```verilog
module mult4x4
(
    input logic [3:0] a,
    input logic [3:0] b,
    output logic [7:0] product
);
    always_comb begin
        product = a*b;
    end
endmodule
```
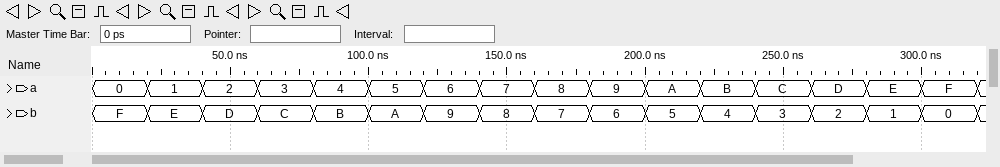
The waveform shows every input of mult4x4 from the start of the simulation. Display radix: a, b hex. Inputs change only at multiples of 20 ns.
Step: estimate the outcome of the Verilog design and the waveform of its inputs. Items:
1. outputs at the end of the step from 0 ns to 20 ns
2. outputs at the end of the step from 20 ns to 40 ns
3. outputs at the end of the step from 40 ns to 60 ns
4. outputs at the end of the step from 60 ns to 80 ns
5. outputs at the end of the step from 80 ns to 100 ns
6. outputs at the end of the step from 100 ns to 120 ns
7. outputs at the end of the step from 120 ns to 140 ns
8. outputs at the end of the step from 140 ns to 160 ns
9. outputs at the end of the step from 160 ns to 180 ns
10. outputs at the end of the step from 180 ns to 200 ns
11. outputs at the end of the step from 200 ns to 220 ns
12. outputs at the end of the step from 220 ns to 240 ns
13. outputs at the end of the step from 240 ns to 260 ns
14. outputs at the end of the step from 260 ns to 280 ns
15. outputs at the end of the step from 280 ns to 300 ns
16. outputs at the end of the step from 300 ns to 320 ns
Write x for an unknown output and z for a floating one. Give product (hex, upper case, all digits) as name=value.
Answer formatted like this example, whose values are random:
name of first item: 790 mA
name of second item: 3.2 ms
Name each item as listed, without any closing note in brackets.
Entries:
outputs at the end of the step from 0 ns to 20 ns: product=00
outputs at the end of the step from 20 ns to 40 ns: product=0E
outputs at the end of the step from 40 ns to 60 ns: product=1A
outputs at the end of the step from 60 ns to 80 ns: product=24
outputs at the end of the step from 80 ns to 100 ns: product=2C
outputs at the end of the step from 100 ns to 120 ns: product=32
outputs at the end of the step from 120 ns to 140 ns: product=36
outputs at the end of the step from 140 ns to 160 ns: product=38
outputs at the end of the step from 160 ns to 180 ns: product=38
outputs at the end of the step from 180 ns to 200 ns: product=36
outputs at the end of the step from 200 ns to 220 ns: product=32
outputs at the end of the step from 220 ns to 240 ns: product=2C
outputs at the end of the step from 240 ns to 260 ns: product=24
outputs at the end of the step from 260 ns to 280 ns: product=1A
outputs at the end of the step from 280 ns to 300 ns: product=0E
outputs at the end of the step from 300 ns to 320 ns: product=00
